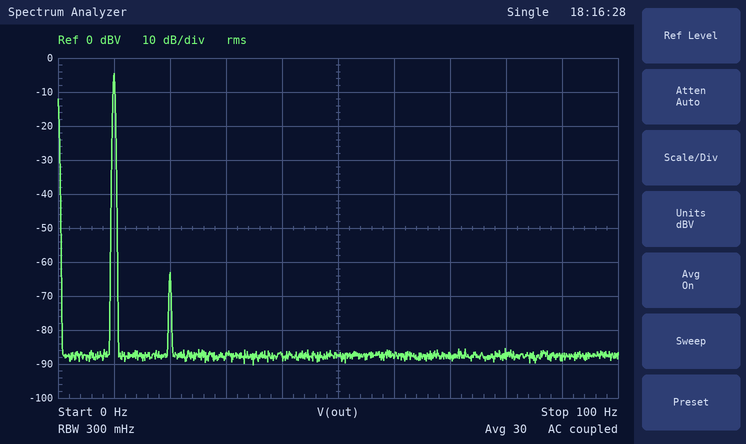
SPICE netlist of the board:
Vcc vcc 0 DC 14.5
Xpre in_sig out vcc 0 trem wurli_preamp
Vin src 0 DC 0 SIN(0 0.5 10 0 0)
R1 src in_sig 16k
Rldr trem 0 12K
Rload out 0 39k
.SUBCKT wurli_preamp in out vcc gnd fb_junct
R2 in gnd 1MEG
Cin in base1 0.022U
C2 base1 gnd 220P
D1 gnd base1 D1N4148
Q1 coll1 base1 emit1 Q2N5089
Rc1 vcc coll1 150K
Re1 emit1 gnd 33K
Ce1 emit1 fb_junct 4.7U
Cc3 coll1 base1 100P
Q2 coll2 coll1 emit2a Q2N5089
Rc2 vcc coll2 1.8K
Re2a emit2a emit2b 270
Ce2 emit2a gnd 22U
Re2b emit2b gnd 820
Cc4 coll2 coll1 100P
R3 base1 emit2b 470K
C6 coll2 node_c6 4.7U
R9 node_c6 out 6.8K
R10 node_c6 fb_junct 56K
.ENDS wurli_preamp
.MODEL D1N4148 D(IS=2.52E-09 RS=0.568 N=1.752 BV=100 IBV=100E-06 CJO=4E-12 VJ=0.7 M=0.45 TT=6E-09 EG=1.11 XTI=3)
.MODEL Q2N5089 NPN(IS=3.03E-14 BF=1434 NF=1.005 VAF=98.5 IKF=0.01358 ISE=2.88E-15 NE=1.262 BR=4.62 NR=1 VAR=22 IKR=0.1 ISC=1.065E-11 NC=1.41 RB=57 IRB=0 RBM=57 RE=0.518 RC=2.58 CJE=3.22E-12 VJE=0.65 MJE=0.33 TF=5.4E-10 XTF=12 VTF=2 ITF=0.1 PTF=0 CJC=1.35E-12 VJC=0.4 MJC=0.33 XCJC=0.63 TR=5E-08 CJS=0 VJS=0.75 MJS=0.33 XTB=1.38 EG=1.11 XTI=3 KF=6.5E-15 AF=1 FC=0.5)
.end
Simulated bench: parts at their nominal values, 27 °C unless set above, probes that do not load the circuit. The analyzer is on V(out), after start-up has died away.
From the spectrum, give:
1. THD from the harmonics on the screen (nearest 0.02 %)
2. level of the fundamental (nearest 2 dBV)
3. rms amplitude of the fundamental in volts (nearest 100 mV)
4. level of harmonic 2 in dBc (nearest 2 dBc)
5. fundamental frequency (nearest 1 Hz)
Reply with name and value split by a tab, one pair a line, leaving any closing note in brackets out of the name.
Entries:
THD from the harmonics on the screen	0.12 %
level of the fundamental	-4 dBV
rms amplitude of the fundamental in volts	600 mV
level of harmonic 2 in dBc	-58 dBc
fundamental frequency	10 Hz
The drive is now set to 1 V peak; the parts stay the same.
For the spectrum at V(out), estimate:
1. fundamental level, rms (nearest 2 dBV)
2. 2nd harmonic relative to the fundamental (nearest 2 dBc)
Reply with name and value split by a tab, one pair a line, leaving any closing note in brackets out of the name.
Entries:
fundamental level, rms	2 dBV
2nd harmonic relative to the fundamental	-52 dBc
